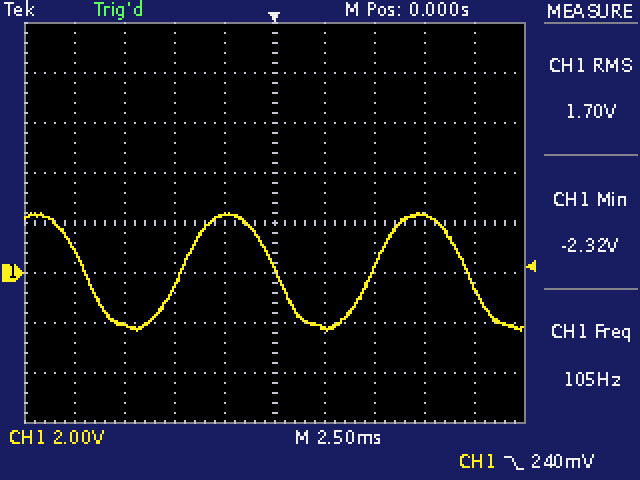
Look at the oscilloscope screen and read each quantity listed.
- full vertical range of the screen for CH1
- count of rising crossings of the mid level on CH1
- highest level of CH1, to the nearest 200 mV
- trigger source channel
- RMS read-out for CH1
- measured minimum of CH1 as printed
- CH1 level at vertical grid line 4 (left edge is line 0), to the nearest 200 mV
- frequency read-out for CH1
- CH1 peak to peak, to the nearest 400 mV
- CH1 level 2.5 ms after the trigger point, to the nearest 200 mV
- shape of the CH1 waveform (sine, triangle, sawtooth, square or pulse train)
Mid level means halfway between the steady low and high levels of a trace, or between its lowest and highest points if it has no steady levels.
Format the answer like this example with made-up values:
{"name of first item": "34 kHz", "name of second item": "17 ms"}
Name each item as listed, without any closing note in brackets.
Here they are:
{"full vertical range of the screen for CH1": "16 V", "count of rising crossings of the mid level on CH1": "2", "highest level of CH1, to the nearest 200 mV": "2.4 V", "trigger source channel": "CH1", "RMS read-out for CH1": "1.70 V", "measured minimum of CH1 as printed": "-2.32 V", "CH1 level at vertical grid line 4 (left edge is line 0), to the nearest 200 mV": "2.4 V", "frequency read-out for CH1": "105 Hz", "CH1 peak to peak, to the nearest 400 mV": "4.8 V", "CH1 level 2.5 ms after the trigger point, to the nearest 200 mV": "-2.2 V", "shape of the CH1 waveform": "sine"}
